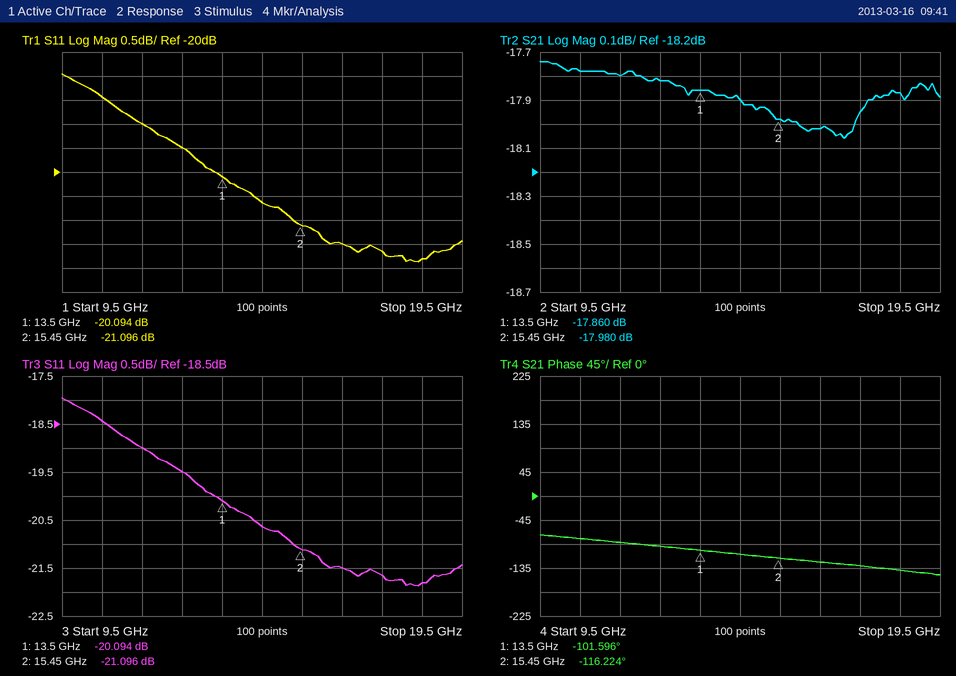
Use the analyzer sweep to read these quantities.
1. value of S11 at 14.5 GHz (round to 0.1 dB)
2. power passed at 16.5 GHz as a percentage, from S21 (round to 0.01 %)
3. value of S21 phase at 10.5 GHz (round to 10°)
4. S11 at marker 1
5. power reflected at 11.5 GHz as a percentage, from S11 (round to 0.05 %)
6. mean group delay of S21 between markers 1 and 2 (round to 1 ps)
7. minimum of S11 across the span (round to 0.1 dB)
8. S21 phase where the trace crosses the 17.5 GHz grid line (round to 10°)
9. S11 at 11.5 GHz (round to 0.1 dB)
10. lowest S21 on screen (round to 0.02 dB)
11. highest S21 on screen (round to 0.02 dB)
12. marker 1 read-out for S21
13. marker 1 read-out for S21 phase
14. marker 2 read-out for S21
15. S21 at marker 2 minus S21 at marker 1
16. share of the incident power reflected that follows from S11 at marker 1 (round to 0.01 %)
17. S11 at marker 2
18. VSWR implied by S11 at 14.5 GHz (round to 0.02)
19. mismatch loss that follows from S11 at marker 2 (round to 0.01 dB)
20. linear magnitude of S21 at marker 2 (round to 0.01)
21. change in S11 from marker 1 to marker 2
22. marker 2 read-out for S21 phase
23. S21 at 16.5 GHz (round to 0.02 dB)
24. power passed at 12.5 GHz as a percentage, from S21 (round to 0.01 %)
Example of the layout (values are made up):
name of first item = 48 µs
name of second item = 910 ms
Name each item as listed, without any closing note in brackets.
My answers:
value of S11 at 14.5 GHz = -20.6 dB
power passed at 16.5 GHz as a percentage, from S21 = 1.58 %
value of S21 phase at 10.5 GHz = -80°
S11 at marker 1 = -20.094 dB
power reflected at 11.5 GHz as a percentage, from S11 = 1.25 %
mean group delay of S21 between markers 1 and 2 = 21 ps
minimum of S11 across the span = -21.9 dB
S21 phase where the trace crosses the 17.5 GHz grid line = -130°
S11 at 11.5 GHz = -19.0 dB
lowest S21 on screen = -18.06 dB
highest S21 on screen = -17.74 dB
marker 1 read-out for S21 = -17.860 dB
marker 1 read-out for S21 phase = -101.596°
marker 2 read-out for S21 = -17.980 dB
S21 at marker 2 minus S21 at marker 1 = -0.120 dB
share of the incident power reflected that follows from S11 at marker 1 = 0.98 %
S11 at marker 2 = -21.096 dB
VSWR implied by S11 at 14.5 GHz = 1.20
mismatch loss that follows from S11 at marker 2 = 0.03 dB
linear magnitude of S21 at marker 2 = 0.13
change in S11 from marker 1 to marker 2 = -1.002 dB
marker 2 read-out for S21 phase = -116.224°
S21 at 16.5 GHz = -18.02 dB
power passed at 12.5 GHz as a percentage, from S21 = 1.65 %
